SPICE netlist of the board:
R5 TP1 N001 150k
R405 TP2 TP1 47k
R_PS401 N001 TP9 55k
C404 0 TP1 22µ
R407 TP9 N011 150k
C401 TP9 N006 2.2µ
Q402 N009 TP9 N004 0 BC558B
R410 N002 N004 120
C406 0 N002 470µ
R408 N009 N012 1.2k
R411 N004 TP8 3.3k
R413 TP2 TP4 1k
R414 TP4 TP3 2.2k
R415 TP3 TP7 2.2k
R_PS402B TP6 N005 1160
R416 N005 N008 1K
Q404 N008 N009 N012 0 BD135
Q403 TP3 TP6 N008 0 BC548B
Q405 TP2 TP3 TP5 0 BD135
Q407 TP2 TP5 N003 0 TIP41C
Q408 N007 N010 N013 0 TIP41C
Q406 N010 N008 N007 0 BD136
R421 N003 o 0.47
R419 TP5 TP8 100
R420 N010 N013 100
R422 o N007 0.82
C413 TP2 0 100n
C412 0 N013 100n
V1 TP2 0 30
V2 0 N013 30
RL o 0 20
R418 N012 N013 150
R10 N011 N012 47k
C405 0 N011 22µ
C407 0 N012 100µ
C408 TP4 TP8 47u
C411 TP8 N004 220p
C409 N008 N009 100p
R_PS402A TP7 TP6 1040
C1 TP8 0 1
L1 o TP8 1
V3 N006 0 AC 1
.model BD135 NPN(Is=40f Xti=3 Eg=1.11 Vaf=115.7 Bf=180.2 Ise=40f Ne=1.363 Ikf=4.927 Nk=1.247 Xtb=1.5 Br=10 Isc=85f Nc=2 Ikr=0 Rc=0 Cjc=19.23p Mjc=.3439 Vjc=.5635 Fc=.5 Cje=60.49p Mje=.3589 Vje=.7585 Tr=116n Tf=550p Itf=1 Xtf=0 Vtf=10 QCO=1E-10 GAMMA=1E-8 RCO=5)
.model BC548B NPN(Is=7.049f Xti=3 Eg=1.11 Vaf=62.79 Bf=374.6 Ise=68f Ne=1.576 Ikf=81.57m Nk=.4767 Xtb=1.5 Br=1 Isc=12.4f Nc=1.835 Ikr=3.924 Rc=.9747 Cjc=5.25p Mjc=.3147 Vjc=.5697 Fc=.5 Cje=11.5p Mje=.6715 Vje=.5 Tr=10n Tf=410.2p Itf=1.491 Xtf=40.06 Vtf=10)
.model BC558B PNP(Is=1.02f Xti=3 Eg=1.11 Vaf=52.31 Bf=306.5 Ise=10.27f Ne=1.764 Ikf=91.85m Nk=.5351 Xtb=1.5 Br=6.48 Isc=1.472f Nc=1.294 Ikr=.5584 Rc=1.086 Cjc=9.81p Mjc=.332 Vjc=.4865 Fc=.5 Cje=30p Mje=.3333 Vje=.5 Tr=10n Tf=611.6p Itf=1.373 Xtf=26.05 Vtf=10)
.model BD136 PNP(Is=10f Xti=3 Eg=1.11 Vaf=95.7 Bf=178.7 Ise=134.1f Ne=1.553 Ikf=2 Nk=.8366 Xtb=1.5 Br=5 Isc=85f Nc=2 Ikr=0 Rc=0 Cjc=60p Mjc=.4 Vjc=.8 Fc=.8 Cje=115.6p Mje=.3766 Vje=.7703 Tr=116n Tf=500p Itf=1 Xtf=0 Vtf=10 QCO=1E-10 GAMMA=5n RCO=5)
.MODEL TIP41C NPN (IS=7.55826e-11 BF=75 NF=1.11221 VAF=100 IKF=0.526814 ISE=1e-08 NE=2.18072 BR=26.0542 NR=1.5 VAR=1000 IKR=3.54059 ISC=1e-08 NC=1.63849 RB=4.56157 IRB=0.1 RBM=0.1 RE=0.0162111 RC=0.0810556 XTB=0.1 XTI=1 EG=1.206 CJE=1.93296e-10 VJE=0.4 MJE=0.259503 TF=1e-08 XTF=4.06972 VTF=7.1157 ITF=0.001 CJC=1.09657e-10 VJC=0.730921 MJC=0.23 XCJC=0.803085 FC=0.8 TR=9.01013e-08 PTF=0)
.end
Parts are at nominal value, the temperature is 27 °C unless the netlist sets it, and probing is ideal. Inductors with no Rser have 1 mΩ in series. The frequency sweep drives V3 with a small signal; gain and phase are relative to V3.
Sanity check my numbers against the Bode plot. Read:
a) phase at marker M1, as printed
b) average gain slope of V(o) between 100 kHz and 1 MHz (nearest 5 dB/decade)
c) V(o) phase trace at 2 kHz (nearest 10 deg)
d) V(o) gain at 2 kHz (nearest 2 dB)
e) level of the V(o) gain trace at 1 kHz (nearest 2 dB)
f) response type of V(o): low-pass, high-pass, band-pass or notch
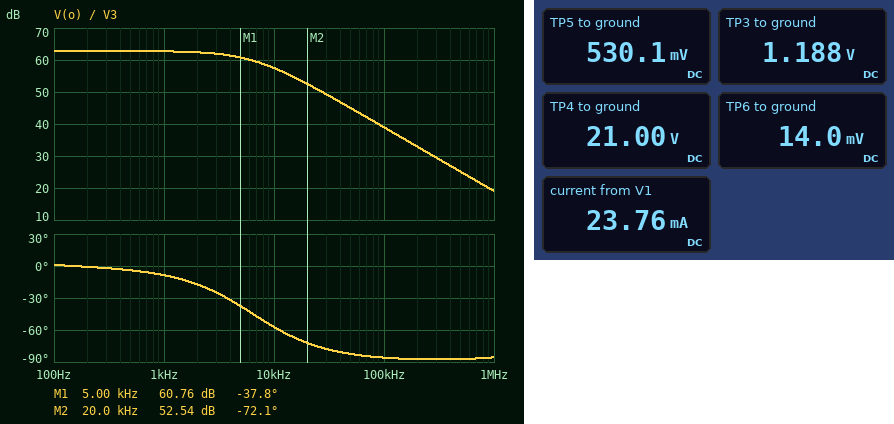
-37.8 deg
-20 dB/decade
-20 deg
62 dB
62 dB
low-pass
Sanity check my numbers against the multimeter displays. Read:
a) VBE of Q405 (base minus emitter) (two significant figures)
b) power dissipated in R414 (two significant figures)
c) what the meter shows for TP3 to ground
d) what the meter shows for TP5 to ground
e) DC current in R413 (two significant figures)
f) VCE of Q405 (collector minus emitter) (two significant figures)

660 mV
180 mW
1.188 V
530.1 mV
9.0 mA
29 V
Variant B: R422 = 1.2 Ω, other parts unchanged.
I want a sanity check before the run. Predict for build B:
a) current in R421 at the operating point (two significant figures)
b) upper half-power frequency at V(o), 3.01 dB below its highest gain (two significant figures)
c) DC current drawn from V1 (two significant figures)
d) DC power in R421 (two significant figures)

8.4 mA
3.0 kHz
23 mA
33 µW
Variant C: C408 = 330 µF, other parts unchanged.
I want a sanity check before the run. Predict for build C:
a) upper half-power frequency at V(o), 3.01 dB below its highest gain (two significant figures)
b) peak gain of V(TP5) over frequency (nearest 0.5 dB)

5.2 kHz
63.5 dB
